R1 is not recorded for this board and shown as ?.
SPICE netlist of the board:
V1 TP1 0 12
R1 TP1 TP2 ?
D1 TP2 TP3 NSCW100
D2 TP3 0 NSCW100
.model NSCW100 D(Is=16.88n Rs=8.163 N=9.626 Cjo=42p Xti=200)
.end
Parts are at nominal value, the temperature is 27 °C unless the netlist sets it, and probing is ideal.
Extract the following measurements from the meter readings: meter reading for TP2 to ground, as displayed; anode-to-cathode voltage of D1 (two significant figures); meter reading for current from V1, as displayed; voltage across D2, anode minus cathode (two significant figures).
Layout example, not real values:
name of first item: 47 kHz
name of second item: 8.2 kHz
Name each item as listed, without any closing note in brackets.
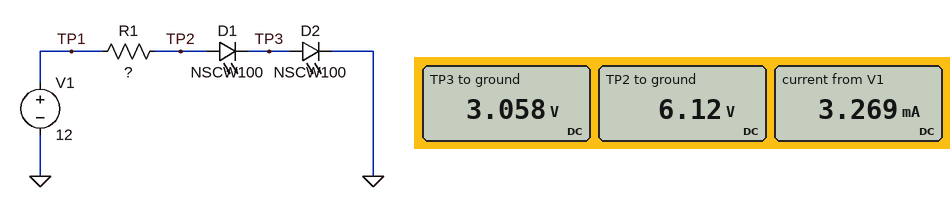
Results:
meter reading for TP2 to ground, as displayed: 6.12 V
anode-to-cathode voltage of D1: 3.1 V
meter reading for current from V1, as displayed: 3.269 mA
voltage across D2, anode minus cathode: 3.1 V
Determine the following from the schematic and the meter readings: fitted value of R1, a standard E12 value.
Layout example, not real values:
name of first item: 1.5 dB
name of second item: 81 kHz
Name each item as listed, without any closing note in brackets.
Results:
fitted value of R1, a standard E12 value: 1.8 kΩ
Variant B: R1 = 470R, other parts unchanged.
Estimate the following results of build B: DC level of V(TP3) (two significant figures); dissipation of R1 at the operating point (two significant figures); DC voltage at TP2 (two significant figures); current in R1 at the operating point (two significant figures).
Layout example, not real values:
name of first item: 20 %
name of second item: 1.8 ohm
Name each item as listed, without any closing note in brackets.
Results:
DC level of V(TP3): 3.4 V
dissipation of R1 at the operating point: 57 mW
DC voltage at TP2: 6.8 V
current in R1 at the operating point: 11 mA
